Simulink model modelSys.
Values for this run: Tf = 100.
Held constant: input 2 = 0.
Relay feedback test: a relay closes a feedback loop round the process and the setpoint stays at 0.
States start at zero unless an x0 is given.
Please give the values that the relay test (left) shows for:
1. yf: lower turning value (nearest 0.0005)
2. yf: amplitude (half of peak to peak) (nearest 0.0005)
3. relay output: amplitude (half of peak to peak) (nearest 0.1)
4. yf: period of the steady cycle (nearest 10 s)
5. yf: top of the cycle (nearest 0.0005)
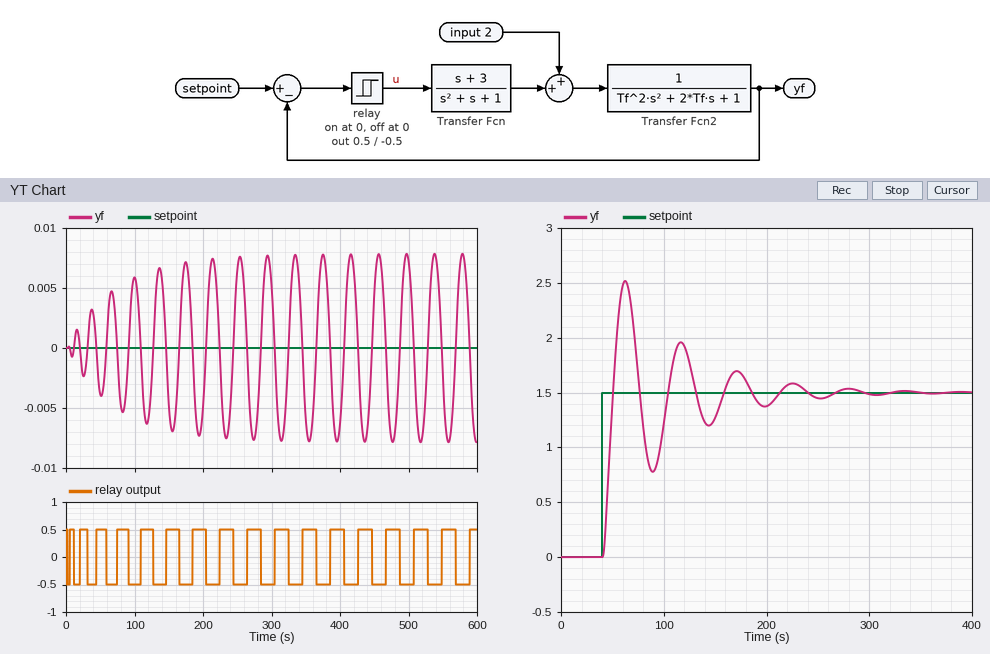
-0.0080
0.0080
0.5
40 s
0.0080
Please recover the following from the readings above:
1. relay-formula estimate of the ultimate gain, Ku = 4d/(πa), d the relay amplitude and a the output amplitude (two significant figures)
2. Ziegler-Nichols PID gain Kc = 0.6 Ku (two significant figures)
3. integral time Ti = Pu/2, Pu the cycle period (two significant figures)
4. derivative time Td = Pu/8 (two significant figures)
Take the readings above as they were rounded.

80
48
20 s
5.0 s
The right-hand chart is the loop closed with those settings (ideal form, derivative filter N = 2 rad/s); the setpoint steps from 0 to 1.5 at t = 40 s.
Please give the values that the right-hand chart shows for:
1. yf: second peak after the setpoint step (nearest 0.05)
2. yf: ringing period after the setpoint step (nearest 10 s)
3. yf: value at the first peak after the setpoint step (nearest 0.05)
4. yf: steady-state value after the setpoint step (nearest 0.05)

1.95
50 s
2.50
1.50
